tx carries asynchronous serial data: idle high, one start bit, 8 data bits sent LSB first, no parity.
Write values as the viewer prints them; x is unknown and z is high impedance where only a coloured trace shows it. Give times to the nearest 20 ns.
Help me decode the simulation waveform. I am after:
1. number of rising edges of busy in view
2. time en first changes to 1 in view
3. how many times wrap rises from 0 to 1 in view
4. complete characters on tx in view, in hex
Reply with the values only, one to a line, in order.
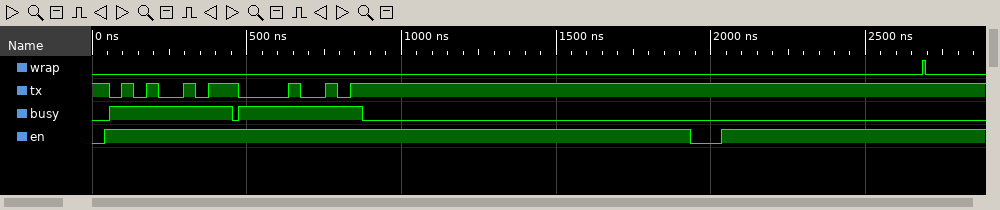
2
40 ns
1
A5, 48
